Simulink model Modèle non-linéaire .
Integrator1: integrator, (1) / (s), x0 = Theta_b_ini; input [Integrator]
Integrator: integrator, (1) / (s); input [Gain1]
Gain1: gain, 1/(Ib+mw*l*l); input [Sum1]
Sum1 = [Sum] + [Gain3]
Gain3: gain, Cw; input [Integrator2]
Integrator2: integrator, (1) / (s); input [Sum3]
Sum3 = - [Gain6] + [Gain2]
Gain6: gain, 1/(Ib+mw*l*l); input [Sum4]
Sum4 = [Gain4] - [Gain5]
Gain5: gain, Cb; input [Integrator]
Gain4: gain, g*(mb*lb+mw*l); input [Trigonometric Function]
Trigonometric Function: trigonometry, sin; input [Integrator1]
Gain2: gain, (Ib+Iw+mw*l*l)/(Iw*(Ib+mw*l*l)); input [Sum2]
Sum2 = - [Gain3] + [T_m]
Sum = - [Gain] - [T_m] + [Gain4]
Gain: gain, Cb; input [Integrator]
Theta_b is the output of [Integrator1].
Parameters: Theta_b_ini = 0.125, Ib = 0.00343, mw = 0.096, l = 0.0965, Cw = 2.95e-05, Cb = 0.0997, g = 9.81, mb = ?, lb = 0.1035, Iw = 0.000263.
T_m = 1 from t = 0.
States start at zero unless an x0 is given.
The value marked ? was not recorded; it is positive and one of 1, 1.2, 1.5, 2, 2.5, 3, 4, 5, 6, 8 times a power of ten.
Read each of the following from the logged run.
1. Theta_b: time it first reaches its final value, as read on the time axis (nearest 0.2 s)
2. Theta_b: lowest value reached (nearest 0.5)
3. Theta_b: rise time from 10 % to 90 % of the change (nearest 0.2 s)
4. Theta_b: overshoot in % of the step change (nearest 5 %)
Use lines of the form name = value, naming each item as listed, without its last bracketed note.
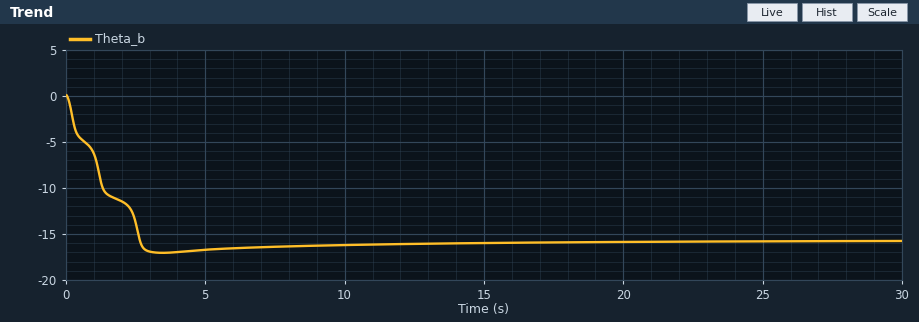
Theta_b: time it first reaches its final value, as read on the time axis = 2.6 s
Theta_b: lowest value reached = -17.0
Theta_b: rise time from 10 % to 90 % of the change = 2.4 s
Theta_b: overshoot in % of the step change = 10 %
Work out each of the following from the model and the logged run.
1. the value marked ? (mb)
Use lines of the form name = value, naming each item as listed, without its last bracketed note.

the value marked ? = 0.6
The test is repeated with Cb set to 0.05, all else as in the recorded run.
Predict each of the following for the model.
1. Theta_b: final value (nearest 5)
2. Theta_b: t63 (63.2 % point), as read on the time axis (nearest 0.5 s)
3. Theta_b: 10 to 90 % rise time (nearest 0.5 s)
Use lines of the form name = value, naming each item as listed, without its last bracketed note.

Theta_b: final value = -55
Theta_b: t63 (63.2 % point), as read on the time axis = 2.0 s
Theta_b: 10 to 90 % rise time = 3.0 s
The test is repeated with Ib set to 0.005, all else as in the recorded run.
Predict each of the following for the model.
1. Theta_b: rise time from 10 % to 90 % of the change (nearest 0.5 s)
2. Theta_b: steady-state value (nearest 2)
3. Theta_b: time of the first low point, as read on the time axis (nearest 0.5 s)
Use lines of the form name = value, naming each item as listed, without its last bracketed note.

Theta_b: rise time from 10 % to 90 % of the change = 2.0 s
Theta_b: steady-state value = -16
Theta_b: time of the first low point, as read on the time axis = 3.5 s
